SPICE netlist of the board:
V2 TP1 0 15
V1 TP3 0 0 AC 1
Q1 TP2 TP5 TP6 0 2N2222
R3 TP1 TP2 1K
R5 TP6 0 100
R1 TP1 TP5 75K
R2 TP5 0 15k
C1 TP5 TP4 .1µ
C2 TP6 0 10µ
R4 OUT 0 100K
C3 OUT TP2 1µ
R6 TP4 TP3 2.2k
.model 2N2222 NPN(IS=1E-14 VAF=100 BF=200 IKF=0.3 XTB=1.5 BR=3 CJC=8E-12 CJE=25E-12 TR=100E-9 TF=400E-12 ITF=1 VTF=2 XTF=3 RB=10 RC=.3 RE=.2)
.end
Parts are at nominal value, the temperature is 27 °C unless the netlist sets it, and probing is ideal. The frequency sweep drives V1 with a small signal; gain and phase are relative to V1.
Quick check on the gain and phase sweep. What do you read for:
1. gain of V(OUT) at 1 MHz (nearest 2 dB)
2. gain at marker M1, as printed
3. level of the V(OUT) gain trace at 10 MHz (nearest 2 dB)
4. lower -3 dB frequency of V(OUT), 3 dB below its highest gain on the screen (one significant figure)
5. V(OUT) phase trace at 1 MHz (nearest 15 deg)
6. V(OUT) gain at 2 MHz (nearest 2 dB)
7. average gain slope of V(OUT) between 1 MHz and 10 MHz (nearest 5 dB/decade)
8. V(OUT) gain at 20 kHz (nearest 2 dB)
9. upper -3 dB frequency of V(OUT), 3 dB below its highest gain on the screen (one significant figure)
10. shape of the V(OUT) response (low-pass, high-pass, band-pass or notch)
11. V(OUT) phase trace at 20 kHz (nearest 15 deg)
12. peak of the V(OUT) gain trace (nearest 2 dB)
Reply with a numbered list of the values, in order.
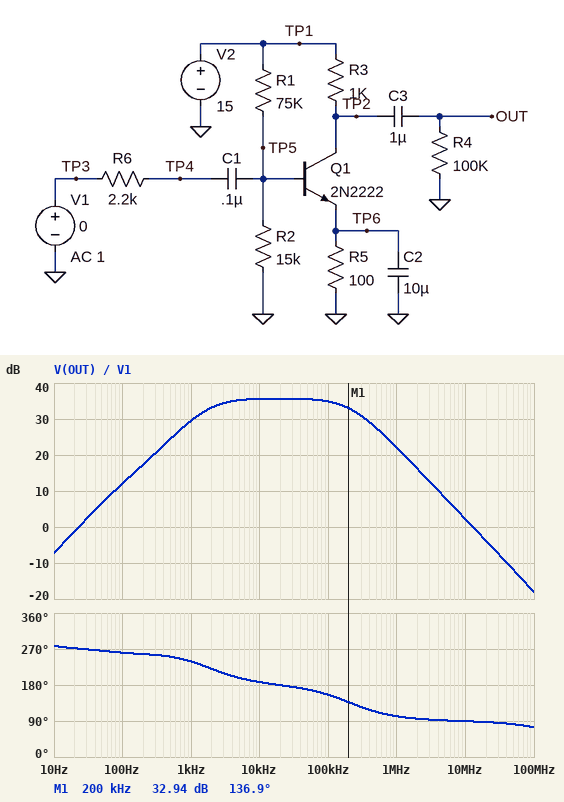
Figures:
1. 22 dB
2. 32.94 dB
3. 2 dB
4. 2 kHz
5. 105 deg
6. 16 dB
7. -20 dB/decade
8. 36 dB
9. 200 kHz
10. band-pass
11. 180 deg
12. 36 dB
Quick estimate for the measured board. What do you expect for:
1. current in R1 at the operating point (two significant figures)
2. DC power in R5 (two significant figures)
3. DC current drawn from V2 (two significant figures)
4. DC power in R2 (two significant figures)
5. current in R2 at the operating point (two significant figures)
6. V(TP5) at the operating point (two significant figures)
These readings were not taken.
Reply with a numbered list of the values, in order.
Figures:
1. 180 µA
2. 12 mW
3. 11 mA
4. 220 µW
5. 120 µA
6. 1.8 V
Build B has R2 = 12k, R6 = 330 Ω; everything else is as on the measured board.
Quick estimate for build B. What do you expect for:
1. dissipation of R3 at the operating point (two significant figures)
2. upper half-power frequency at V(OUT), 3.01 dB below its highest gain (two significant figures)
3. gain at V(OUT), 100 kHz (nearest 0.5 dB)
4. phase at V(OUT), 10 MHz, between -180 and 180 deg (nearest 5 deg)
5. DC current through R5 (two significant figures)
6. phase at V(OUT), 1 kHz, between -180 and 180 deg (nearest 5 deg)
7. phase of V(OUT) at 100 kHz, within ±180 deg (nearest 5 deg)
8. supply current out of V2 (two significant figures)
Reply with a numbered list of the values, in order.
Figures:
1. 80 mW
2. 540 kHz
3. 45.0 dB
4. 90 deg
5. 9.0 mA
6. -100 deg
7. 170 deg
8. 9.1 mA
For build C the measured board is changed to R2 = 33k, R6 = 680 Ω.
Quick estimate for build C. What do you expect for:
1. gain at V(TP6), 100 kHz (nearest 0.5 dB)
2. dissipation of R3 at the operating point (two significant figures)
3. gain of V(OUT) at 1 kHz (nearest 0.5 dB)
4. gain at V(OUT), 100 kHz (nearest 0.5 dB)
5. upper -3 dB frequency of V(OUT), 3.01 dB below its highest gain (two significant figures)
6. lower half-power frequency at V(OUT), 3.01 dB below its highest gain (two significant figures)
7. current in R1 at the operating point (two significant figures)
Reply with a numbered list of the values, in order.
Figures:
1. -68.5 dB
2. 180 mW
3. -8.5 dB
4. -0.5 dB
5. 530 kHz
6. 2.3 kHz
7. 170 µA
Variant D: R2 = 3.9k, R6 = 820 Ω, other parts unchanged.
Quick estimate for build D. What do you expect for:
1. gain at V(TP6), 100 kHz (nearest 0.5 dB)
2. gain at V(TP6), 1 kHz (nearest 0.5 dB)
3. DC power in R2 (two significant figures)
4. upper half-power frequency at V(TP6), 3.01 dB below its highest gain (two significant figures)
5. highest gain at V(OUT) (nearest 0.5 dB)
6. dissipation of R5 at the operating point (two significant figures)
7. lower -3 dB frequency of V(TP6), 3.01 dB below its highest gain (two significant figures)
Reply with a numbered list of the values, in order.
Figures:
1. -48.5 dB
2. -11.0 dB
3. 140 µW
4. 1.3 kHz
5. 27.0 dB
6. 66 µW
7. 180 Hz
